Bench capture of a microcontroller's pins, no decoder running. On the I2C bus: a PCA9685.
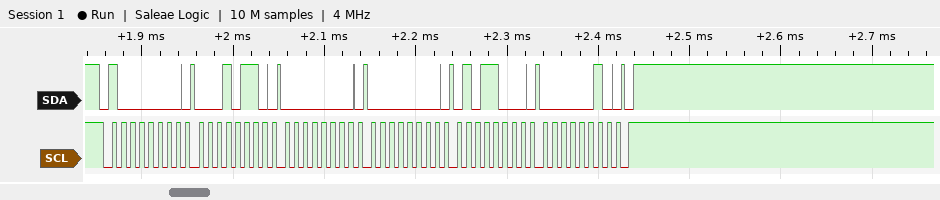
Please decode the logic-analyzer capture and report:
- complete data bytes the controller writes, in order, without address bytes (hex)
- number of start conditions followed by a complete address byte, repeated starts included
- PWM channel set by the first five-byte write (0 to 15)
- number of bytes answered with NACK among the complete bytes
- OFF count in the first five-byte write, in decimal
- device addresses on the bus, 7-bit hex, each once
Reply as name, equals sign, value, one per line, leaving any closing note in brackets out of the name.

complete data bytes the controller writes, in order, without address bytes = 16 00 00 58 02
number of start conditions followed by a complete address byte, repeated starts included = 1
PWM channel set by the first five-byte write = 4
number of bytes answered with NACK among the complete bytes = 0
OFF count in the first five-byte write, in decimal = 600
device addresses on the bus, 7-bit hex, each once = 0x40
